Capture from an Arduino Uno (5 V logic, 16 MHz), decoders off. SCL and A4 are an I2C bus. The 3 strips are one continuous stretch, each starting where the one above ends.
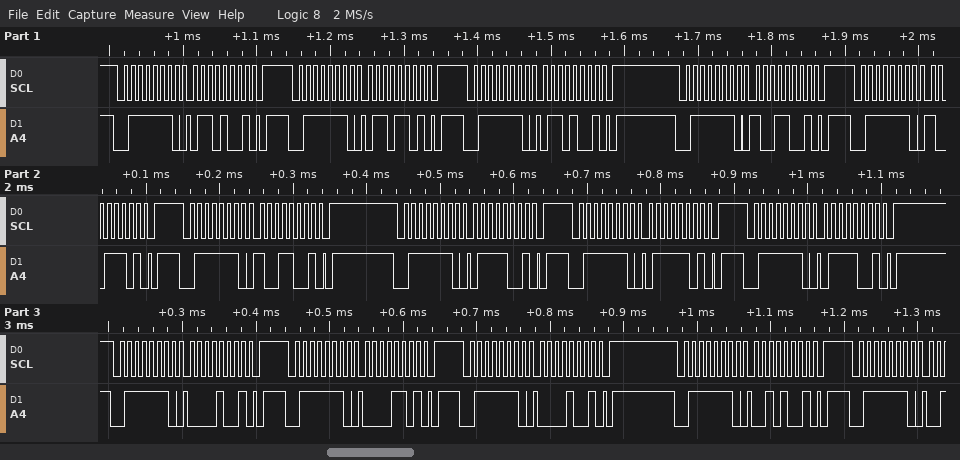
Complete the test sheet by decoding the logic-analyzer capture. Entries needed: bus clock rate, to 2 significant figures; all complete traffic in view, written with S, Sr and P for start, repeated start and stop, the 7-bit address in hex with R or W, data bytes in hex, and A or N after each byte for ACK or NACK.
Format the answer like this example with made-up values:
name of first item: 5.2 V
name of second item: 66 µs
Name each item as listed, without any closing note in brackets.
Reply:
bus clock rate, to 2 significant figures: 100 kHz
all complete traffic in view, written with S, Sr and P for start, repeated start and stop, the 7-bit address in hex with R or W, data bytes in hex, and A or N after each byte for ACK or NACK: S 3FW A 69 A P S 3FW A 6D A P S 3FW A 69 A P S 3FW A 99 A P S 3FW A 9D A P S 3FW A 99 A P S 3FW A 79 A P S 3FW A 7D A P S 3FW A 79 A P S 3FW A 09 A P S 3FW A 0D A P S 3FW A 09 A P S 3FW A 29 A P S 3FW A
